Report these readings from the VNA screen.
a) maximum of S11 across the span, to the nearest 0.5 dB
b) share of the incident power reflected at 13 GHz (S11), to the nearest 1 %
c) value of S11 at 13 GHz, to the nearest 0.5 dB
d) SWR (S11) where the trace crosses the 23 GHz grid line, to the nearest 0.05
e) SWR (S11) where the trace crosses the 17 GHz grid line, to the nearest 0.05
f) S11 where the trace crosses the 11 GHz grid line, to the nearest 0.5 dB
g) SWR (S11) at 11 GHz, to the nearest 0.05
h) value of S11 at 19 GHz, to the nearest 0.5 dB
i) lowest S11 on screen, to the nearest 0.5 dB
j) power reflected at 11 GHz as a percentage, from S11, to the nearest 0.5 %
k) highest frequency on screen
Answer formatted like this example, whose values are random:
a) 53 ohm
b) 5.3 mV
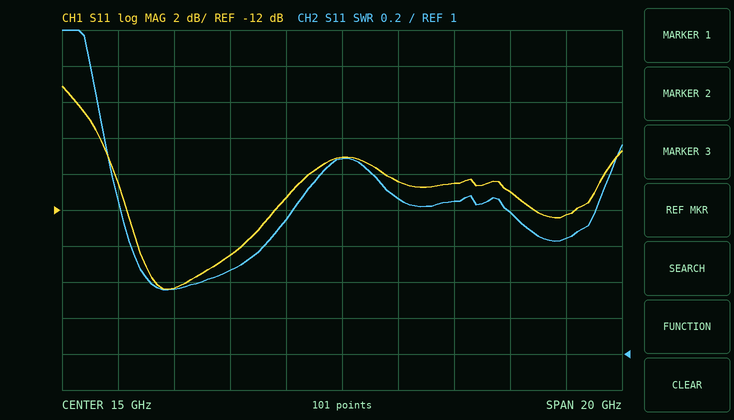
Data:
a) -5.0 dB
b) 7 %
c) -11.5 dB
d) 1.65
e) 1.85
f) -14.5 dB
g) 1.45
h) -10.5 dB
i) -16.5 dB
j) 3.5 %
k) 25 GHz
